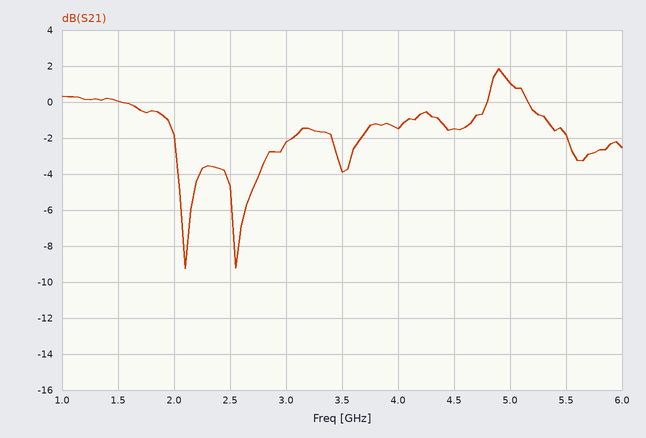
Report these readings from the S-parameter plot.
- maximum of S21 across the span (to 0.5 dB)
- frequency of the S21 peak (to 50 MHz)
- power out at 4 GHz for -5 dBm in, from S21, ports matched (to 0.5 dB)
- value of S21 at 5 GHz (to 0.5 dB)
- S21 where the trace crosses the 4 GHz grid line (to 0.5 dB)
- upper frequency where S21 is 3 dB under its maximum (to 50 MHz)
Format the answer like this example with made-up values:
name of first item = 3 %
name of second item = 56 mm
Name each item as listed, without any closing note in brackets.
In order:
maximum of S21 across the span = 2.0 dB
frequency of the S21 peak = 4.90 GHz
power out at 4 GHz for -5 dBm in, from S21, ports matched = -6.5 dBm
value of S21 at 5 GHz = 1.0 dB
S21 where the trace crosses the 4 GHz grid line = -1.5 dB
upper frequency where S21 is 3 dB under its maximum = 5.35 GHz
